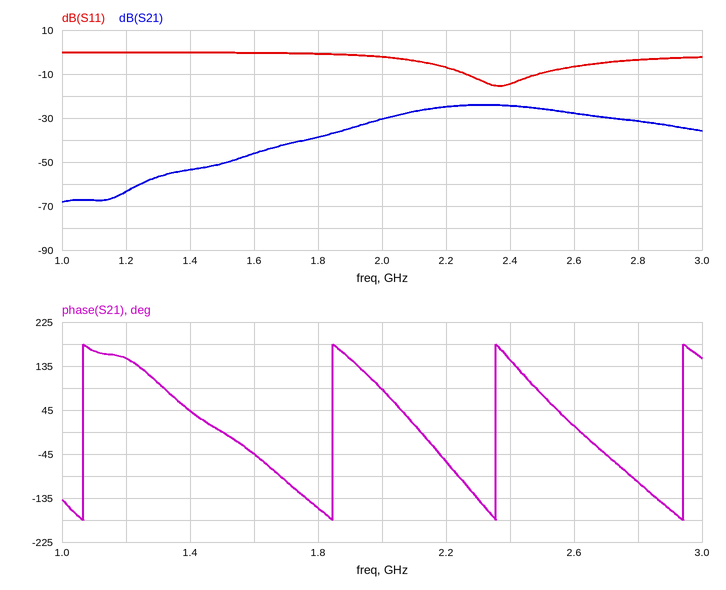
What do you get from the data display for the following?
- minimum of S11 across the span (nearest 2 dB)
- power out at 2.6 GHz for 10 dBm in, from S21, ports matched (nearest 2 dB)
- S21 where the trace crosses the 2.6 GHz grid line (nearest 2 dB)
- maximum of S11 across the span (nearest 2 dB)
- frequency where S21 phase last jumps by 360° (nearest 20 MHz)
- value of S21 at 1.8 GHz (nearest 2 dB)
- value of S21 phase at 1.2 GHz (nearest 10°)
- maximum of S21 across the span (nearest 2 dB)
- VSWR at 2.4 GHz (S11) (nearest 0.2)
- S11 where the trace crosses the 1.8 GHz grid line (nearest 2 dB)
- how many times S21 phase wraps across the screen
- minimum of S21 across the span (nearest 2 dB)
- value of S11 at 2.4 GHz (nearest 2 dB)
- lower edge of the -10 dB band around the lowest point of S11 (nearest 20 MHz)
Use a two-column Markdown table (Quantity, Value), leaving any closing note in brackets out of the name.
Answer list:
| Quantity | Value |
|---|---|
| minimum of S11 across the span | -16 dB |
| power out at 2.6 GHz for 10 dBm in, from S21, ports matched | -18 dBm |
| S21 where the trace crosses the 2.6 GHz grid line | -28 dB |
| maximum of S11 across the span | 0 dB |
| frequency where S21 phase last jumps by 360° | 2.94 GHz |
| value of S21 at 1.8 GHz | -38 dB |
| value of S21 phase at 1.2 GHz | 150° |
| maximum of S21 across the span | -24 dB |
| VSWR at 2.4 GHz (S11) | 1.4 |
| S11 where the trace crosses the 1.8 GHz grid line | 0 dB |
| how many times S21 phase wraps across the screen | 4 |
| minimum of S21 across the span | -68 dB |
| value of S11 at 2.4 GHz | -14 dB |
| lower edge of the -10 dB band around the lowest point of S11 | 2.26 GHz |
